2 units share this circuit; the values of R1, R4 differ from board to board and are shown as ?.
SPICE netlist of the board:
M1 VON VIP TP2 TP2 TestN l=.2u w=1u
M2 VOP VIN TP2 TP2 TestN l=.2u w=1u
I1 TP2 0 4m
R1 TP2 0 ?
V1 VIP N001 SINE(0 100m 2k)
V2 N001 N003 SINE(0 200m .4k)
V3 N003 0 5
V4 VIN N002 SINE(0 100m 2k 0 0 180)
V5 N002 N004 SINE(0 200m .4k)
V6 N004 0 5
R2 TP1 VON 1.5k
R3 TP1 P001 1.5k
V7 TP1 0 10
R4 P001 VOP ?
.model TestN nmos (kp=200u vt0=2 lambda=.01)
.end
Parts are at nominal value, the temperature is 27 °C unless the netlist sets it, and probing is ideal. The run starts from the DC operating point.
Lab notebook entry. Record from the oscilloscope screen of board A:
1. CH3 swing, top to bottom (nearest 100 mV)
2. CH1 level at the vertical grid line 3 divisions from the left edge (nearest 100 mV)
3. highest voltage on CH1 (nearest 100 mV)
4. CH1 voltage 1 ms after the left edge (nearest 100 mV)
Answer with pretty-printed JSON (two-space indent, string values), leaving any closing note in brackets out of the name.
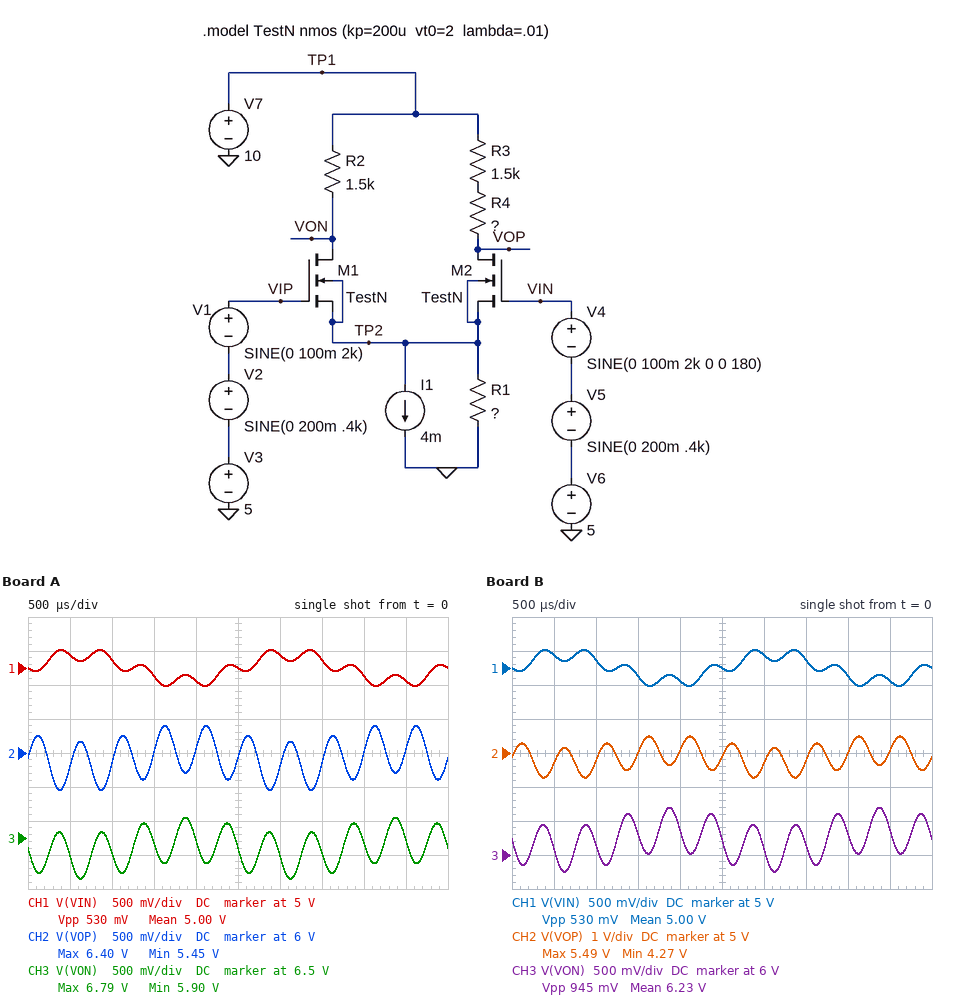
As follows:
{
  "CH3 swing, top to bottom": "900 mV",
  "CH1 level at the vertical grid line 3 divisions from the left edge": "4.9 V",
  "highest voltage on CH1": "5.3 V",
  "CH1 voltage 1 ms after the left edge": "5.1 V"
}
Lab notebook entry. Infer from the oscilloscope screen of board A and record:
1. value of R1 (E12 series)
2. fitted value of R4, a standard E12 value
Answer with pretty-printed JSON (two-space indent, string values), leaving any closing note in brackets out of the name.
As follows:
{
  "value of R1": "1 kΩ",
  "fitted value of R4, a standard E12 value": "180 Ω"
}
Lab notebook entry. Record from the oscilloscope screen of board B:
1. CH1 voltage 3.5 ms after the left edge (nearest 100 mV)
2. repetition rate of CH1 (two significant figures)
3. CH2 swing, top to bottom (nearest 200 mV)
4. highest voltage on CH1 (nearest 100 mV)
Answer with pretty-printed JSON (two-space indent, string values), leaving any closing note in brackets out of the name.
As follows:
{
  "CH1 voltage 3.5 ms after the left edge": "5.1 V",
  "repetition rate of CH1": "400 Hz",
  "CH2 swing, top to bottom": "1.2 V",
  "highest voltage on CH1": "5.3 V"
}
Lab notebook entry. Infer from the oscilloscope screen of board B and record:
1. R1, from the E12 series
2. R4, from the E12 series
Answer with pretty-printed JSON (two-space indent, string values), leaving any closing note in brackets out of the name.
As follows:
{
  "R1, from the E12 series": "820 Ω",
  "R4, from the E12 series": "560 Ω"
}
